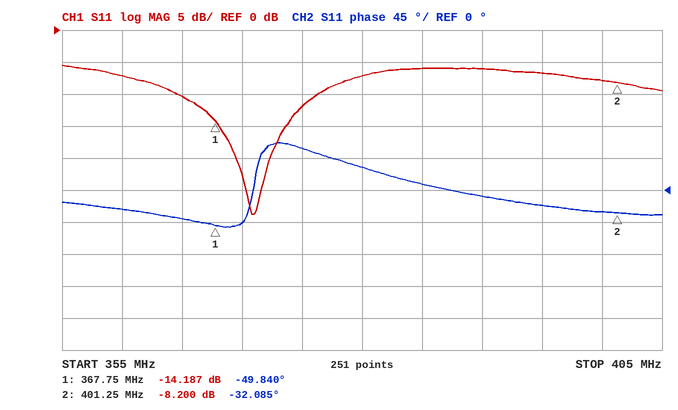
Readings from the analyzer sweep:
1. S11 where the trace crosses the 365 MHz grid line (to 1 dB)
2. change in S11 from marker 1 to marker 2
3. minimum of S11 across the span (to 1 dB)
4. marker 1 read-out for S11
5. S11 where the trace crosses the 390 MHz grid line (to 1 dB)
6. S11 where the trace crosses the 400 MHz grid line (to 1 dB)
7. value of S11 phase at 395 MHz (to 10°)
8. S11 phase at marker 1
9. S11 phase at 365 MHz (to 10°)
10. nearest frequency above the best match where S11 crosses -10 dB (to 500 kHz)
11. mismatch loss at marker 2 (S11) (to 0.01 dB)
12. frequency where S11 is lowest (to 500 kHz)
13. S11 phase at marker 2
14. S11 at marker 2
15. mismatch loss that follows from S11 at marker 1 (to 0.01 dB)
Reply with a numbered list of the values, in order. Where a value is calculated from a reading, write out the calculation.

1. -10 dB
2. -8.2 − (-14.187) = 5.987 dB
3. -29 dB
4. -14.187 dB
5. -6 dB
6. -8 dB
7. -20°
8. -49.840°
9. -40°
10. 376.5 MHz
11. −10 log10(1 − 10^(-8.2/10)) ≈ 0.71 dB
12. 371.0 MHz
13. -32.085°
14. -8.200 dB
15. −10 log10(1 − 10^(-14.187/10)) ≈ 0.17 dB
